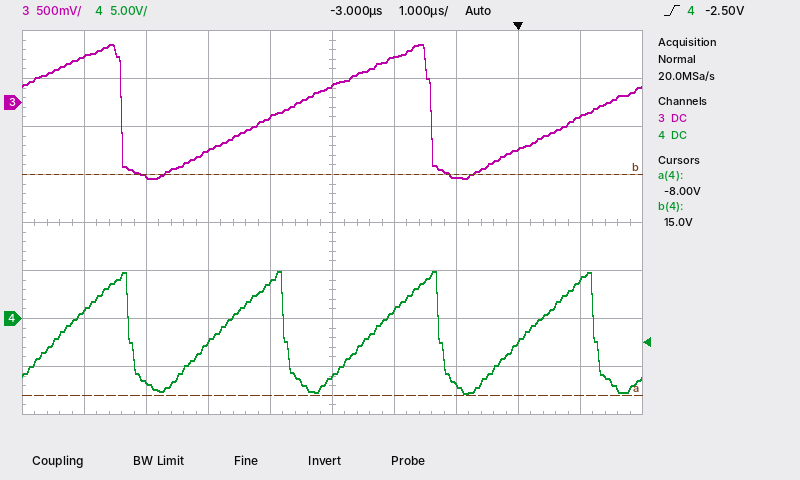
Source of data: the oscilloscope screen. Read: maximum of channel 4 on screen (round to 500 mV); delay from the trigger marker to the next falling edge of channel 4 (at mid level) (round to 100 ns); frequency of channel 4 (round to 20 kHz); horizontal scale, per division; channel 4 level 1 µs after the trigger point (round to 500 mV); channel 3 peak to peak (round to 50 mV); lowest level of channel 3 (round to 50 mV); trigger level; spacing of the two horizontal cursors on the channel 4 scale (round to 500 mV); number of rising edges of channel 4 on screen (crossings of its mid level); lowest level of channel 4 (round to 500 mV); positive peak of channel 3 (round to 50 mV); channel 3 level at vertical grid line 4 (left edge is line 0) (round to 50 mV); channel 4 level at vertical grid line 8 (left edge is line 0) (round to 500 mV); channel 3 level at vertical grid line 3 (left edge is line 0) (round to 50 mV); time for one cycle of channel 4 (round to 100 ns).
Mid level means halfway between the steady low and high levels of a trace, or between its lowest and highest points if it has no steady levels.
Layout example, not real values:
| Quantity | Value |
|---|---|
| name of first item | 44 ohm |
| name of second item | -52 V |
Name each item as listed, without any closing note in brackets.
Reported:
| Quantity | Value |
|---|---|
| maximum of channel 4 on screen | 5.0 V |
| delay from the trigger marker to the next falling edge of channel 4 (at mid level) | 1.2 µs |
| frequency of channel 4 | 400 kHz |
| horizontal scale, per division | 1 µs |
| channel 4 level 1 µs after the trigger point | 4.0 V |
| channel 3 peak to peak | 1.40 V |
| lowest level of channel 3 | -800 mV |
| trigger level | -2.50 V |
| spacing of the two horizontal cursors on the channel 4 scale | 23.0 V |
| number of rising edges of channel 4 on screen | 4 |
| lowest level of channel 4 | -8.0 V |
| positive peak of channel 3 | 600 mV |
| channel 3 level at vertical grid line 4 (left edge is line 0) | -150 mV |
| channel 4 level at vertical grid line 8 (left edge is line 0) | -2.5 V |
| channel 3 level at vertical grid line 3 (left edge is line 0) | -500 mV |
| time for one cycle of channel 4 | 2.5 µs |
